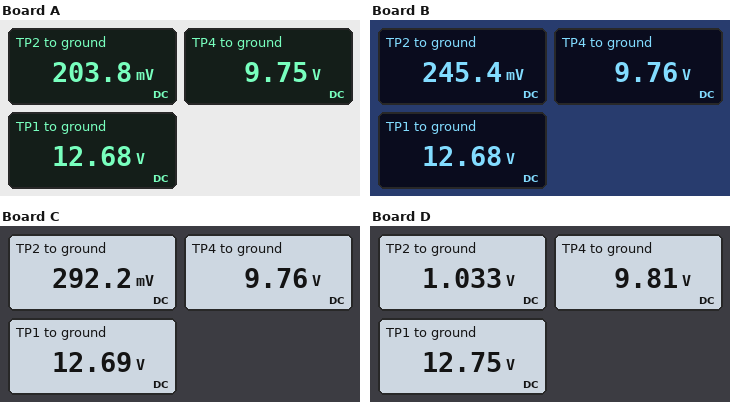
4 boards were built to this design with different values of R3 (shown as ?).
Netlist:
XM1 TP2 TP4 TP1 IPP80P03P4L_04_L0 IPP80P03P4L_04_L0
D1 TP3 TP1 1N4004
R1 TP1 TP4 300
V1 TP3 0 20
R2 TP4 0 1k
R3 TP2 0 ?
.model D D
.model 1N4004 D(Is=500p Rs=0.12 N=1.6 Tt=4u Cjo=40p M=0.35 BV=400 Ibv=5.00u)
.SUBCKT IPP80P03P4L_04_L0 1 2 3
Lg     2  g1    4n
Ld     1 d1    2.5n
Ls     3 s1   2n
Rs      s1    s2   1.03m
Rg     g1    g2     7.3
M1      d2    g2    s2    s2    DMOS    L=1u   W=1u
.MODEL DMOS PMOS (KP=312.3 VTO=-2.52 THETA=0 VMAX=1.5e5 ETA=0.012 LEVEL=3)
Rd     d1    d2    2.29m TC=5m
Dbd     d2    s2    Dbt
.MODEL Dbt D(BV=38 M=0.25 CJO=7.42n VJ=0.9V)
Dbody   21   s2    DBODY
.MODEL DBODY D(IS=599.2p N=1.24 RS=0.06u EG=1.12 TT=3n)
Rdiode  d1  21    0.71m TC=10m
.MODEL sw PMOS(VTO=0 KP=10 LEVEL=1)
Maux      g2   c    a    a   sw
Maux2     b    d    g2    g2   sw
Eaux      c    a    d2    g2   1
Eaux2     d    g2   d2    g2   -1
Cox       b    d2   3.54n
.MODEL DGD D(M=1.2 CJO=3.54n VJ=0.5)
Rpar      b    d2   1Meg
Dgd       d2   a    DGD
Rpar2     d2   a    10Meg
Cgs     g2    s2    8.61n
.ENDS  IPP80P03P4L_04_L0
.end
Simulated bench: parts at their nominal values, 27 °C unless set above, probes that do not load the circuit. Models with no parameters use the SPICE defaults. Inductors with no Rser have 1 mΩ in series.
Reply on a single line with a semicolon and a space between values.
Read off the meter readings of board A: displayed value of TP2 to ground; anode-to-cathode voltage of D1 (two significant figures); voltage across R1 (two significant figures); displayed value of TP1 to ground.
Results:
203.8 mV; 7.3 V; 2.9 V; 12.68 V
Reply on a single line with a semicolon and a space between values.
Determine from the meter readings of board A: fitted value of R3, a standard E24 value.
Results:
3.9 mΩ
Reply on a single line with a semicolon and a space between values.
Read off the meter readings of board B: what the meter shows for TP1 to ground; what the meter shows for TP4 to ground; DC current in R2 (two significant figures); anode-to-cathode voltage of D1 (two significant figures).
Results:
12.68 V; 9.76 V; 9.8 mA; 7.3 V
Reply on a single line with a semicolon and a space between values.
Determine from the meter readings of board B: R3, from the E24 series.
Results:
4.7 mΩ
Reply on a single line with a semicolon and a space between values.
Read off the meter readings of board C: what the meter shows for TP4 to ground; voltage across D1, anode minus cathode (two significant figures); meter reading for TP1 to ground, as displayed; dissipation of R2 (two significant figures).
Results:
9.76 V; 7.3 V; 12.69 V; 95 mW
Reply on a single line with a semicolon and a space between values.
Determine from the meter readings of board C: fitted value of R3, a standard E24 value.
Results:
5.6 mΩ
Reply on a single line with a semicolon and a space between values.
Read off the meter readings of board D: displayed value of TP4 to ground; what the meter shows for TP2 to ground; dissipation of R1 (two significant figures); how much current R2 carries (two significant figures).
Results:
9.81 V; 1.033 V; 29 mW; 9.8 mA
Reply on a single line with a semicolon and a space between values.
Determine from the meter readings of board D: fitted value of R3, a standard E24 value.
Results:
0.02 Ω
